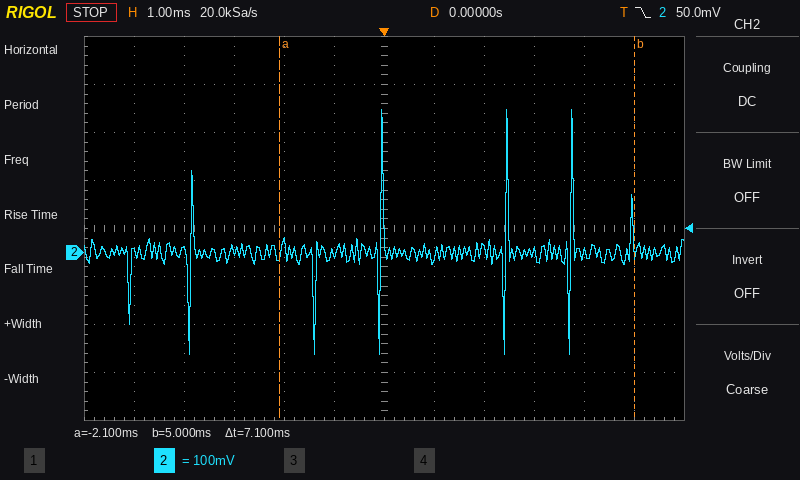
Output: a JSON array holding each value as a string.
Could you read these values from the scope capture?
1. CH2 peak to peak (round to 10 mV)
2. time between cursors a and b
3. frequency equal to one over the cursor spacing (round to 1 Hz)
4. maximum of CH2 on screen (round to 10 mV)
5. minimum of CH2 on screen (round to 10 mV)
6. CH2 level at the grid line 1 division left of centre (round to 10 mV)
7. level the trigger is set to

["510 mV", "7.1 ms", "141 Hz", "300 mV", "-210 mV", "0 mV", "50.0 mV"]
